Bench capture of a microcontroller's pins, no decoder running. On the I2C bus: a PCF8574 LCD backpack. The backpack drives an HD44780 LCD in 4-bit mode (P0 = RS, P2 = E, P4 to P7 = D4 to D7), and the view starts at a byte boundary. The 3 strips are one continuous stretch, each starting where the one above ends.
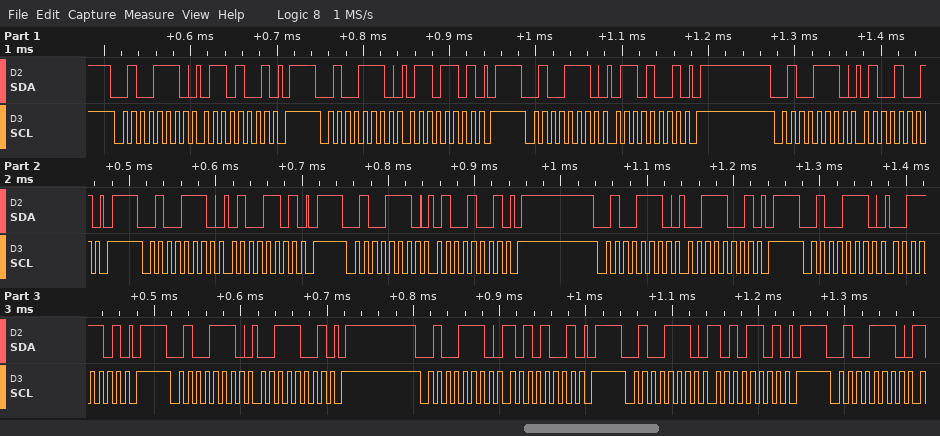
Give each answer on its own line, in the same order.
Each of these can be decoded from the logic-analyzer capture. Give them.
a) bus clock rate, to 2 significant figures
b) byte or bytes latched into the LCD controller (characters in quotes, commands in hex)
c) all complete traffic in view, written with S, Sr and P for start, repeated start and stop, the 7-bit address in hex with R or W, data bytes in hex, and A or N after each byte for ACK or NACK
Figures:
100 kHz
'd'
S 27W A 69 A P S 27W A 6D A P S 27W A 69 A P S 27W A 49 A P S 27W A 4D A P S 27W A 49 A P S 27W A 39 A P S 27W A 3D A P S 27W A 39 A P S 27W A A9 A P S 27W A AD A P S 27W A
